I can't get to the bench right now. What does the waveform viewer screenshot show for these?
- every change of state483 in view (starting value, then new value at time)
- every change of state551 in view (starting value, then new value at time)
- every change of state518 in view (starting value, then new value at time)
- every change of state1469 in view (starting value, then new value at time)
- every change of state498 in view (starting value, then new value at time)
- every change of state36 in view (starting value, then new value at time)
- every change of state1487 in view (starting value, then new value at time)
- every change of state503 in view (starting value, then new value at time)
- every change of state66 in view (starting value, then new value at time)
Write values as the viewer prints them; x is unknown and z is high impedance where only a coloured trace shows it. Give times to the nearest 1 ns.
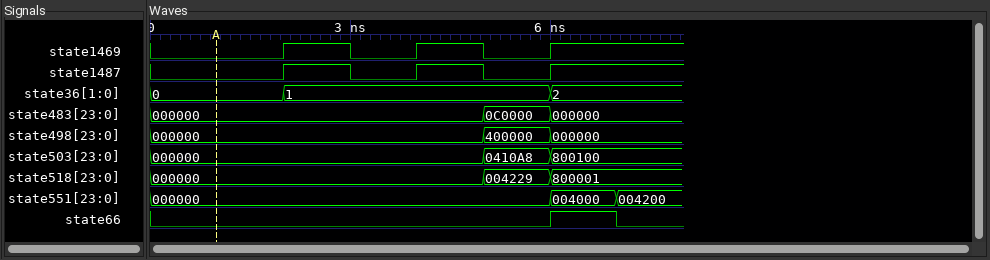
000000, 0C0000 at 5 ns, 000000 at 6 ns
000000, 004000 at 6 ns, 004200 at 7 ns
000000, 004229 at 5 ns, 800001 at 6 ns
0, 1 at 2 ns, 0 at 3 ns, 1 at 4 ns, 0 at 5 ns, 1 at 6 ns
000000, 400000 at 5 ns, 000000 at 6 ns
0, 1 at 2 ns, 2 at 6 ns
0, 1 at 2 ns, 0 at 3 ns, 1 at 4 ns, 0 at 5 ns, 1 at 6 ns
000000, 0410A8 at 5 ns, 800100 at 6 ns
0, 1 at 6 ns, 0 at 7 ns
